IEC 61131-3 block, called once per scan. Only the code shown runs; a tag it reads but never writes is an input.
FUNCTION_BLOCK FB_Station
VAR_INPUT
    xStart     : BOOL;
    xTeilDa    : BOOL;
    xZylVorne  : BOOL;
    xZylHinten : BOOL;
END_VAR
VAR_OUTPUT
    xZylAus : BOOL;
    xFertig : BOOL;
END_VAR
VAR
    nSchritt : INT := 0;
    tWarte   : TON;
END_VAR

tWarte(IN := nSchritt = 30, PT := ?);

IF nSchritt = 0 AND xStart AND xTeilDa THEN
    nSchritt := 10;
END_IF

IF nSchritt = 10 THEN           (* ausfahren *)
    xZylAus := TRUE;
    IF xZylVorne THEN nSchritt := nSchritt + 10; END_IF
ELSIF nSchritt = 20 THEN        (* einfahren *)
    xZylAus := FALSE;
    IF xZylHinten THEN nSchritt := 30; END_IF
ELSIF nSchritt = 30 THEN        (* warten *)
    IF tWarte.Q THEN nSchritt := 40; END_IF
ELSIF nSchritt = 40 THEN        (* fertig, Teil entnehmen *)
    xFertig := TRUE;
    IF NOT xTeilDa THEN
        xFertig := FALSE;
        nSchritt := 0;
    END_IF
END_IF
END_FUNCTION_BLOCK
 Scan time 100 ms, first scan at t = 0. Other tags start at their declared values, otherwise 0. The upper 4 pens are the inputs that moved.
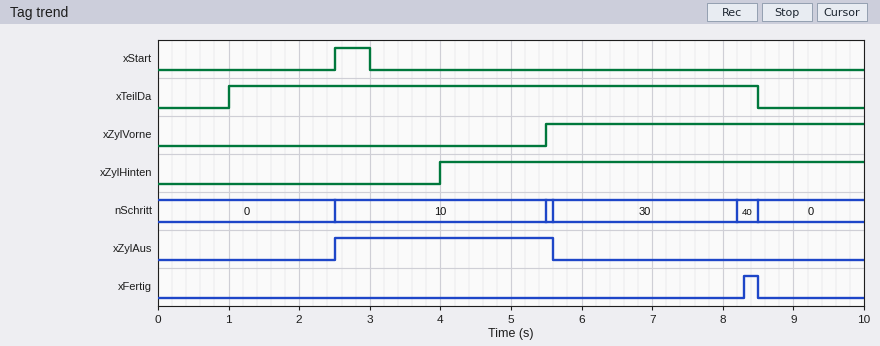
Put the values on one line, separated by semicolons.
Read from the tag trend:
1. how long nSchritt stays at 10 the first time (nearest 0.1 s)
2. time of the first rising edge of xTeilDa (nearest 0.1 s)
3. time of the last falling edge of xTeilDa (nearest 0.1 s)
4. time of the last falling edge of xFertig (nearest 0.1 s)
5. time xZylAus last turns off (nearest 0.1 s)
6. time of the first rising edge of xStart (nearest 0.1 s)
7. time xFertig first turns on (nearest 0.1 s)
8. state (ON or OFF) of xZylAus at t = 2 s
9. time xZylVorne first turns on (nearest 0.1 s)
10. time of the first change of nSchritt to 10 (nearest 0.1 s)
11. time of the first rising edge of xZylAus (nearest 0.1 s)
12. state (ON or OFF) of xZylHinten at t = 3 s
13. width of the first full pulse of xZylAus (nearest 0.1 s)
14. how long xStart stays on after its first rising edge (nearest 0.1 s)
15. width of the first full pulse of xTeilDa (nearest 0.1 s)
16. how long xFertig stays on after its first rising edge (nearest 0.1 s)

3.0 s; 1.0 s; 8.5 s; 8.5 s; 5.6 s; 2.5 s; 8.3 s; OFF; 5.5 s; 2.5 s; 2.5 s; OFF; 3.1 s; 0.5 s; 7.5 s; 0.2 s
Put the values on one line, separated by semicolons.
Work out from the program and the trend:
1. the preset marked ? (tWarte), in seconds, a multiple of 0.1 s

2.5 s
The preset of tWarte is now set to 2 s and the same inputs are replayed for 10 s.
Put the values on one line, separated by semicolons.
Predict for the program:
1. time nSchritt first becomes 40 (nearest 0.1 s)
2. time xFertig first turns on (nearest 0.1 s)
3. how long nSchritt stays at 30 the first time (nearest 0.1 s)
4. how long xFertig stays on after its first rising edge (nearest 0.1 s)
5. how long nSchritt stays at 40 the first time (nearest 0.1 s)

7.7 s; 7.8 s; 2.1 s; 0.7 s; 0.8 s
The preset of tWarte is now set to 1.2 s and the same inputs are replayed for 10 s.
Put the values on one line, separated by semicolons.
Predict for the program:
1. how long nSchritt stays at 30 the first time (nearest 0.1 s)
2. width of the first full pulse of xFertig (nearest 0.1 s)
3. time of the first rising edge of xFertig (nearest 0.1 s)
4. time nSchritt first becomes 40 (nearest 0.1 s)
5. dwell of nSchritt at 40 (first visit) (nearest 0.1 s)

1.3 s; 1.5 s; 7.0 s; 6.9 s; 1.6 s
